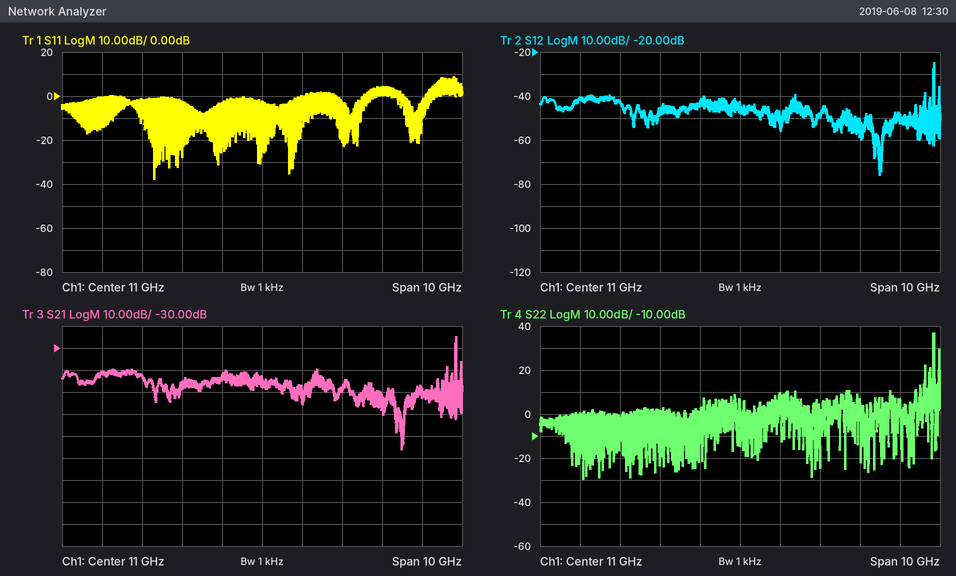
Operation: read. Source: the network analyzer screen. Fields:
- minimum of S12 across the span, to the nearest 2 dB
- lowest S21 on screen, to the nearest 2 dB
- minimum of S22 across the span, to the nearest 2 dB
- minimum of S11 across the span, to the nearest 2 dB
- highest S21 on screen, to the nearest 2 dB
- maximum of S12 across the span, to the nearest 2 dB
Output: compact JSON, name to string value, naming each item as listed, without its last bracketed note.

{"minimum of S12 across the span, to the nearest 2 dB": "-76 dB", "lowest S21 on screen, to the nearest 2 dB": "-76 dB", "minimum of S22 across the span, to the nearest 2 dB": "-30 dB", "minimum of S11 across the span, to the nearest 2 dB": "-38 dB", "highest S21 on screen, to the nearest 2 dB": "-24 dB", "maximum of S12 across the span, to the nearest 2 dB": "-24 dB"}
